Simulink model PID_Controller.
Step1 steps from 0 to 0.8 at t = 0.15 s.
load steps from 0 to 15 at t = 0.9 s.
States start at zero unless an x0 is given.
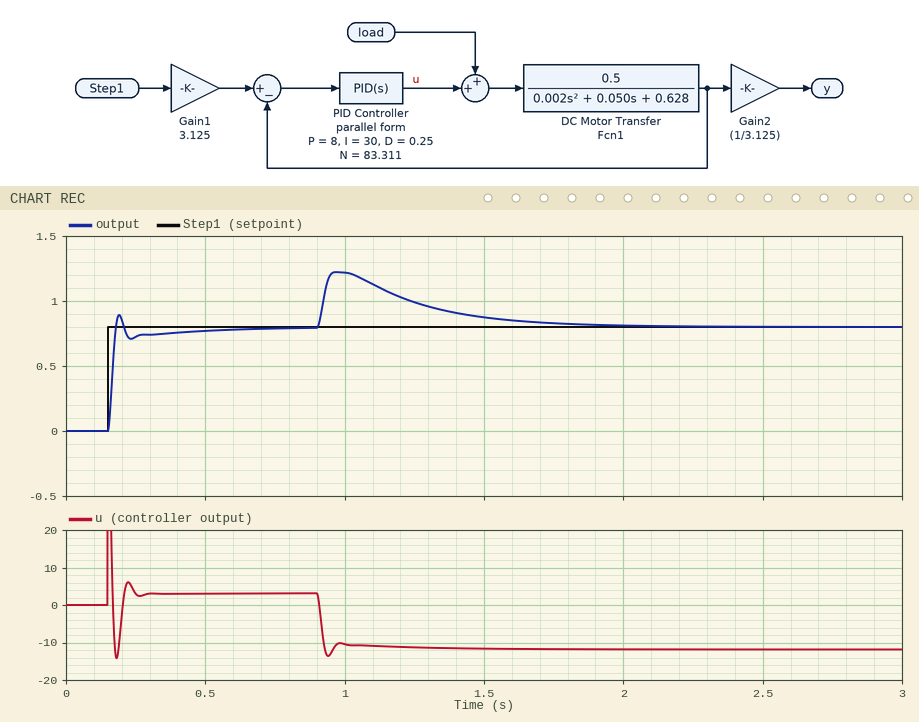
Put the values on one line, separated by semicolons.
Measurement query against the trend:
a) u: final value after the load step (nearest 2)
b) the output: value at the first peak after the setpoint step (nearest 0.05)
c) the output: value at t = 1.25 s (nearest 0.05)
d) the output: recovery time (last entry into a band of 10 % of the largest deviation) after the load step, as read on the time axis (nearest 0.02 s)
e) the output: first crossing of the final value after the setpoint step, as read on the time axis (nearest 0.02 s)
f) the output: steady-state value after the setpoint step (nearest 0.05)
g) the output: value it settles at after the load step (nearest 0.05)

-12; 0.90; 1.00; 1.64 s; 0.18 s; 0.80; 0.80
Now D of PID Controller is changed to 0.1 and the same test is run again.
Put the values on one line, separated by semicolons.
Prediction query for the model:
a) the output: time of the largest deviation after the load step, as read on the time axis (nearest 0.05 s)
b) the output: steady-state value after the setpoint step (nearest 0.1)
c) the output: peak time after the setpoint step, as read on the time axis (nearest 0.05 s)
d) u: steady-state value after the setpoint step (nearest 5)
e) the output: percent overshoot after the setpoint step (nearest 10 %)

0.95 s; 0.8; 0.20 s; 5; 20 %
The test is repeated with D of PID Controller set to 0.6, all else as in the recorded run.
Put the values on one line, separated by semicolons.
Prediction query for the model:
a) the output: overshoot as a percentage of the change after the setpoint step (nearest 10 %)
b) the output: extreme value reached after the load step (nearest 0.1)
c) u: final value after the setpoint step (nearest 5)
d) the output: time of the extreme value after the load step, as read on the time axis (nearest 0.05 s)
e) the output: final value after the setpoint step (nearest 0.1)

20 %; 1.2; 5; 1.05 s; 0.8
